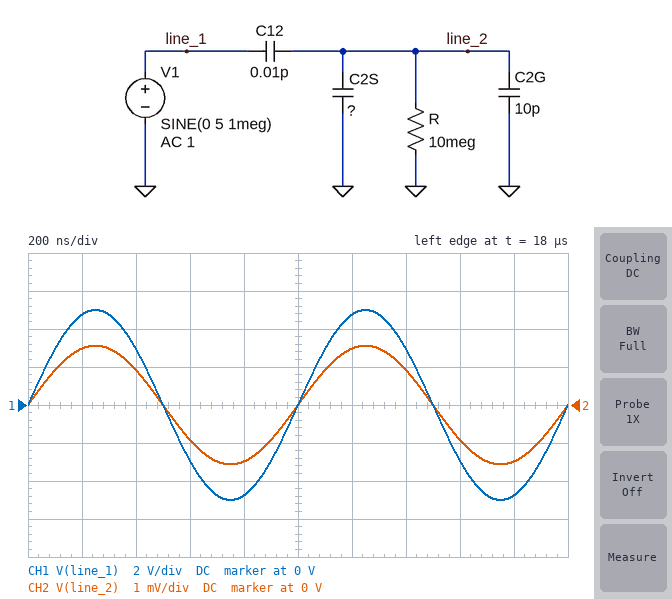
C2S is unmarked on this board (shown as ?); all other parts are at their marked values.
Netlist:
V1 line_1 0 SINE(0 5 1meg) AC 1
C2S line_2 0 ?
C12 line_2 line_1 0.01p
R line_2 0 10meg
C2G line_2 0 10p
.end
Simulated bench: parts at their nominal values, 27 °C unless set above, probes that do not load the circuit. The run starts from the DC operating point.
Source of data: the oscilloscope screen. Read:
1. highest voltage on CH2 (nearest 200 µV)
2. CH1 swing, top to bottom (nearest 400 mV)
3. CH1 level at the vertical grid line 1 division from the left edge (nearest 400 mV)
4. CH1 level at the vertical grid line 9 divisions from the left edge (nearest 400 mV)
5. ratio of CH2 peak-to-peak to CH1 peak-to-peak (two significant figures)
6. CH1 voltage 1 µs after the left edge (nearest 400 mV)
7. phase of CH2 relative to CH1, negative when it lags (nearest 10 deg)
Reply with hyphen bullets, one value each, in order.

- 1.6 mV
- 10.0 V
- 4.8 V
- -4.8 V
- 0.00031
- 0 V
- 0 deg
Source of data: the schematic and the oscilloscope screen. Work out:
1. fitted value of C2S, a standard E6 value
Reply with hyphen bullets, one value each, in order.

- 22 pF
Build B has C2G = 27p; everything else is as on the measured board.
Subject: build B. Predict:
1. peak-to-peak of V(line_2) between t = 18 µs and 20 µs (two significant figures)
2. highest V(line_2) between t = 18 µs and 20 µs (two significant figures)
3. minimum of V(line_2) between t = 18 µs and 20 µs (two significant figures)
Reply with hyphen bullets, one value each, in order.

- 2.0 mV
- 1.0 mV
- -1.0 mV
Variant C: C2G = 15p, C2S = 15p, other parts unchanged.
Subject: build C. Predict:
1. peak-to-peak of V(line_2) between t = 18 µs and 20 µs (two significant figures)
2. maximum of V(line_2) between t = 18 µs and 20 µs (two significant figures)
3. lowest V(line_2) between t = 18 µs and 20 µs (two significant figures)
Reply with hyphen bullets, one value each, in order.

- 3.3 mV
- 1.7 mV
- -1.7 mV
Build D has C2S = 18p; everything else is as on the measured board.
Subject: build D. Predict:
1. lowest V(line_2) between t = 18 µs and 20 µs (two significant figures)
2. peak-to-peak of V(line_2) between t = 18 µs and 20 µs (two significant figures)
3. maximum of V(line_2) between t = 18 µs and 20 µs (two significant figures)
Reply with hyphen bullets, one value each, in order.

- -1.8 mV
- 3.6 mV
- 1.8 mV
